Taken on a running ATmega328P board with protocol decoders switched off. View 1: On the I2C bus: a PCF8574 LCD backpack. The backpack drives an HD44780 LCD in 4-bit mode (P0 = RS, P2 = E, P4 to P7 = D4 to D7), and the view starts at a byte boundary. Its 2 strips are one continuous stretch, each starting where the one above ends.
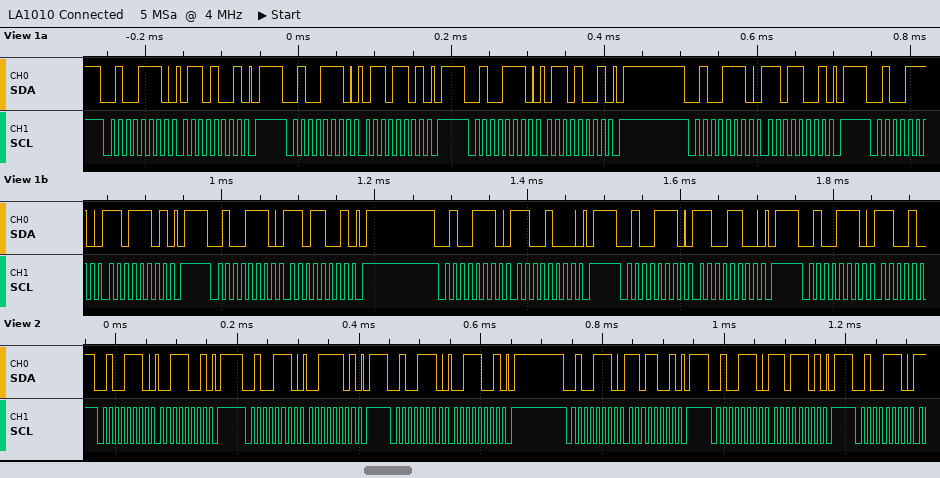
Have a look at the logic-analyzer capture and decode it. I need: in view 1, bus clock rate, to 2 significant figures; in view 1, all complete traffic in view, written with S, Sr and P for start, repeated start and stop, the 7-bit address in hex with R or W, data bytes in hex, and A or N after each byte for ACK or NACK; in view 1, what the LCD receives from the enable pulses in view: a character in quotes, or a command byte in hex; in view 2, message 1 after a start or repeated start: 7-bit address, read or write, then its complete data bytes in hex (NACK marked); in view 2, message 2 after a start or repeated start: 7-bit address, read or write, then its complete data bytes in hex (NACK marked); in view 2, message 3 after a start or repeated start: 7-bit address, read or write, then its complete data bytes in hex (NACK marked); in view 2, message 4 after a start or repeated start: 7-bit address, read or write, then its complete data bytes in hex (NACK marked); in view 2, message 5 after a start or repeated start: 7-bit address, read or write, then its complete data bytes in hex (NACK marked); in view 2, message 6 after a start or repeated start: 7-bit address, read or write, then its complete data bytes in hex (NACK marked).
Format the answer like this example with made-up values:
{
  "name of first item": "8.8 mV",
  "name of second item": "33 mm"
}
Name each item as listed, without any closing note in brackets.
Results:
{
  "in view 1, bus clock rate, to 2 significant figures": "100 kHz",
  "in view 1, all complete traffic in view, written with S, Sr and P for start, repeated start and stop, the 7-bit address in hex with R or W, data bytes in hex, and A or N after each byte for ACK or NACK": "S 27W A 69 A P S 27W A 6D A P S 27W A 69 A P S 27W A D9 A P S 27W A DD A P S 27W A D9 A P S 27W A C8 A P S 27W A CC A P S 27W A",
  "in view 1, what the LCD receives from the enable pulses in view: a character in quotes, or a command byte in hex": "'m'",
  "in view 2, message 1 after a start or repeated start: 7-bit address, read or write, then its complete data bytes in hex": "0x27 write: 39",
  "in view 2, message 2 after a start or repeated start: 7-bit address, read or write, then its complete data bytes in hex": "0x27 write: 3D",
  "in view 2, message 3 after a start or repeated start: 7-bit address, read or write, then its complete data bytes in hex": "0x27 write: 39",
  "in view 2, message 4 after a start or repeated start: 7-bit address, read or write, then its complete data bytes in hex": "0x27 write: D9",
  "in view 2, message 5 after a start or repeated start: 7-bit address, read or write, then its complete data bytes in hex": "0x27 write: DD",
  "in view 2, message 6 after a start or repeated start: 7-bit address, read or write, then its complete data bytes in hex": "0x27 write"
}
